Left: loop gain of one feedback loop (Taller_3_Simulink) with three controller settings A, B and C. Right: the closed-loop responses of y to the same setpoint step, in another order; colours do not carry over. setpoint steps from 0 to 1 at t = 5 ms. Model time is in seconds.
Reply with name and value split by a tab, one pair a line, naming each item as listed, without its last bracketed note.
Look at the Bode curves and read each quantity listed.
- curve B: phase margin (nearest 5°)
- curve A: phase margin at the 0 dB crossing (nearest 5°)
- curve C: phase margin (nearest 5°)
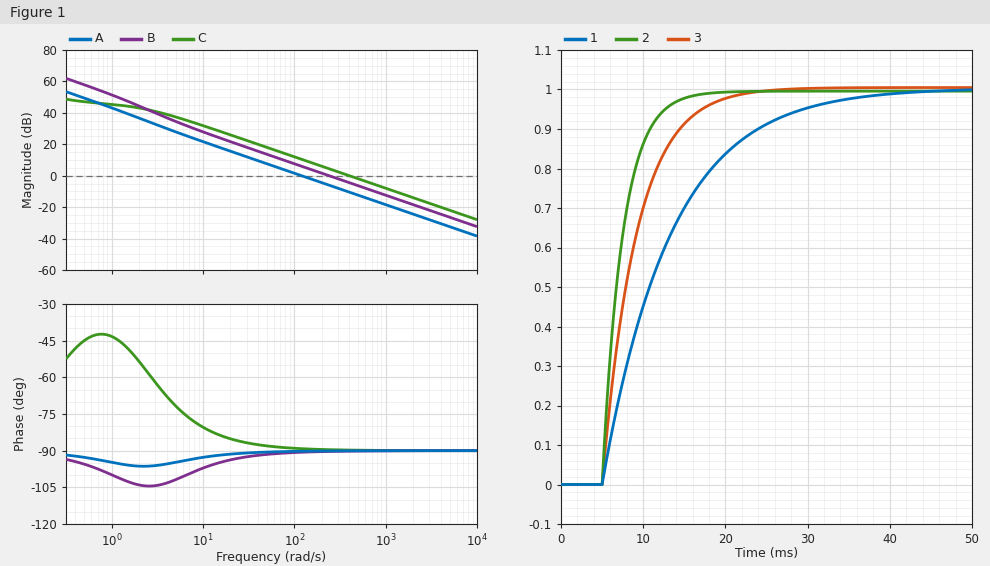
curve B: phase margin	90°
curve A: phase margin at the 0 dB crossing	90°
curve C: phase margin	90°
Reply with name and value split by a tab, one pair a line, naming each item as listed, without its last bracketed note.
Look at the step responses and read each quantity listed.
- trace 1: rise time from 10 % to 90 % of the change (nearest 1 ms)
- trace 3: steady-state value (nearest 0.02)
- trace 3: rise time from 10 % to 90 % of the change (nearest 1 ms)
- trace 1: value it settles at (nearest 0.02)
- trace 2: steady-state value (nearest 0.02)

trace 1: rise time from 10 % to 90 % of the change	18 ms
trace 3: steady-state value	1.00
trace 3: rise time from 10 % to 90 % of the change	9 ms
trace 1: value it settles at	1.00
trace 2: steady-state value	1.00
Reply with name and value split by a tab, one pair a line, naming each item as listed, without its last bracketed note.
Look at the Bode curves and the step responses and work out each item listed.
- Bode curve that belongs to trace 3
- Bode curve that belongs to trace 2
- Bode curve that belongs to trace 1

Bode curve that belongs to trace 3	B
Bode curve that belongs to trace 2	C
Bode curve that belongs to trace 1	A
